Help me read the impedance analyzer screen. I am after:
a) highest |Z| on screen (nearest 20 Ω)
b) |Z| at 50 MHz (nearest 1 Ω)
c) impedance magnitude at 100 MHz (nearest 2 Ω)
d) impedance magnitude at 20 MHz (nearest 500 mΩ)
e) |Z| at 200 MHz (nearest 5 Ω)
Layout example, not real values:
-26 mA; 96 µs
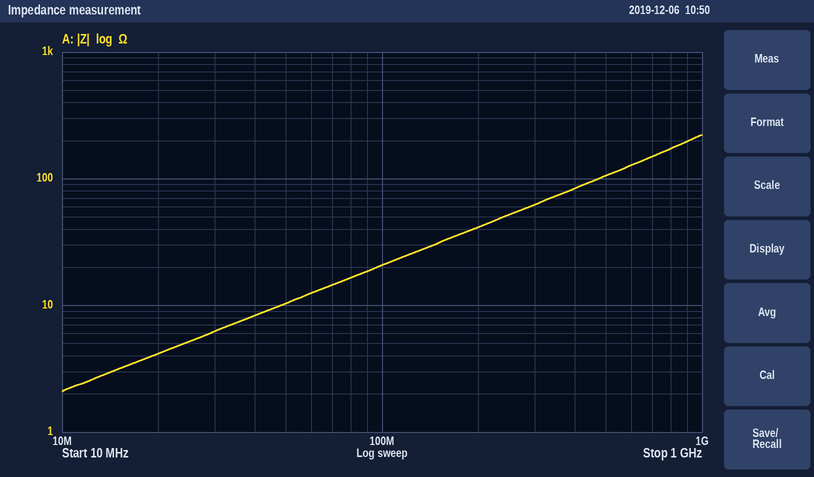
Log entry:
220 Ω; 10 Ω; 20 Ω; 4.0 Ω; 40 Ω
